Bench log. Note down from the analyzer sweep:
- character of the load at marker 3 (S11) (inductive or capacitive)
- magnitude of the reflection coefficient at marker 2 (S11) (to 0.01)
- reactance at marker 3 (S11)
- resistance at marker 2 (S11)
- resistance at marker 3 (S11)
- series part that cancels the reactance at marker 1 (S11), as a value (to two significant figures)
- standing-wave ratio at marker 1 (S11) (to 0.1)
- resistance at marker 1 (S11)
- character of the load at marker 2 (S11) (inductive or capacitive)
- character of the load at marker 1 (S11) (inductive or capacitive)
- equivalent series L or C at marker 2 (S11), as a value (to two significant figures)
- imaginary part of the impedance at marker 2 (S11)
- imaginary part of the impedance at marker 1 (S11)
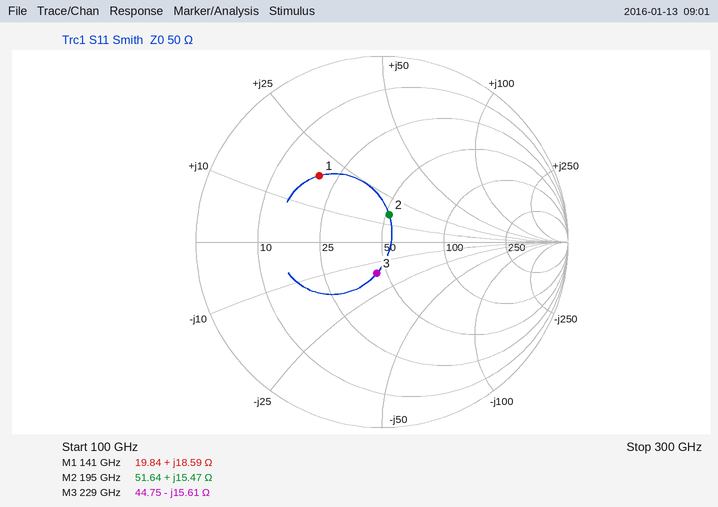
capacitive
0.15
-15.61 Ω
51.64 Ω
44.75 Ω
61 fF
2.9
19.84 Ω
inductive
inductive
13 pH
+15.47 Ω
+18.59 Ω
